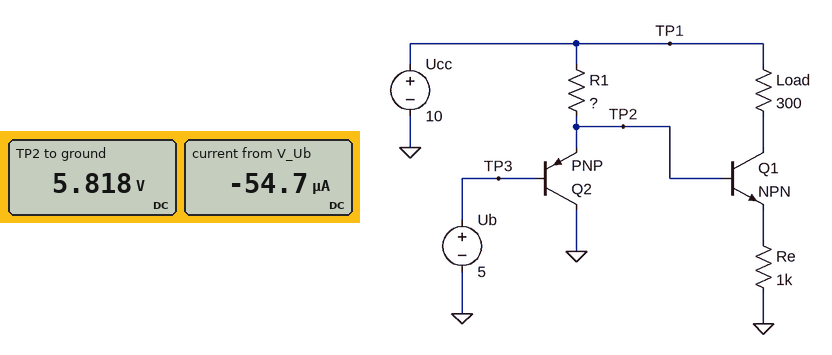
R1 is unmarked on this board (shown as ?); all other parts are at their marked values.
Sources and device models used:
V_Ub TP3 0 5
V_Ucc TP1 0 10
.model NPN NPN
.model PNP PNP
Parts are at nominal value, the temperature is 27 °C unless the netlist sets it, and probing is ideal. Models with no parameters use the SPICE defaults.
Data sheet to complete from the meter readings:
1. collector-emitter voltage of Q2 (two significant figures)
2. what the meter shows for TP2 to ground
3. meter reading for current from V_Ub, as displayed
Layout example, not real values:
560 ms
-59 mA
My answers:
-5.8 V
5.818 V
-54.7 µA
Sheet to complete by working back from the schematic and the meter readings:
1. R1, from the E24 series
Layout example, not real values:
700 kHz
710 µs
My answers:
750 Ω
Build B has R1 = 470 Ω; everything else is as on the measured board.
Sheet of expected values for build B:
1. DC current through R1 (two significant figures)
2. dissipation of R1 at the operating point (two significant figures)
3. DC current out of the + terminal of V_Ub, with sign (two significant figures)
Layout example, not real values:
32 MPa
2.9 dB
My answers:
8.9 mA
37 mW
-87 µA
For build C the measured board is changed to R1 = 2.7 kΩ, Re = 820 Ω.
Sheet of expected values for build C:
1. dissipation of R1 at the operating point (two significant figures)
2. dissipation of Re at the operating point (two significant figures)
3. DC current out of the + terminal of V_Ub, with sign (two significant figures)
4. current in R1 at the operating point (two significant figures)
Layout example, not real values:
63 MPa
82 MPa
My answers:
6.6 mW
30 mW
-15 µA
1.6 mA
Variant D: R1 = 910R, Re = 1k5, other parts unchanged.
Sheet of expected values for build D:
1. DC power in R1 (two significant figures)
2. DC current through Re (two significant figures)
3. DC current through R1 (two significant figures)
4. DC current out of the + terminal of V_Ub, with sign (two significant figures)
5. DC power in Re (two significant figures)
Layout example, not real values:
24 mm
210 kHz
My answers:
19 mW
3.3 mA
4.6 mA
-45 µA
17 mW
